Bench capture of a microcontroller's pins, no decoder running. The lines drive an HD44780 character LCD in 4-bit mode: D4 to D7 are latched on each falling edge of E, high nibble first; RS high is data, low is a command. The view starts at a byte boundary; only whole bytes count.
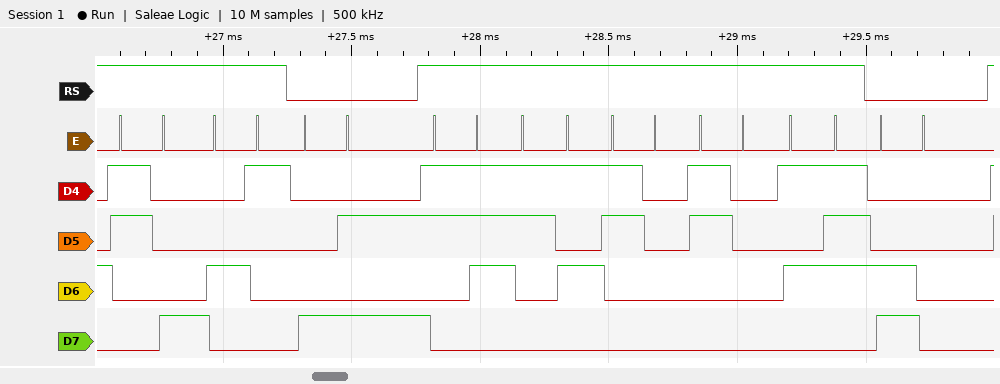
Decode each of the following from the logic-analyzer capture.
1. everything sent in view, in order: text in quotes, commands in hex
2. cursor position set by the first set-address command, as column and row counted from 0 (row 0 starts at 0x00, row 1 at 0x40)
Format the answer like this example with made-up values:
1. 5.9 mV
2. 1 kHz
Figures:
1. "8A" 0x8A "7500W" 0xC0
2. column 10, row 0
